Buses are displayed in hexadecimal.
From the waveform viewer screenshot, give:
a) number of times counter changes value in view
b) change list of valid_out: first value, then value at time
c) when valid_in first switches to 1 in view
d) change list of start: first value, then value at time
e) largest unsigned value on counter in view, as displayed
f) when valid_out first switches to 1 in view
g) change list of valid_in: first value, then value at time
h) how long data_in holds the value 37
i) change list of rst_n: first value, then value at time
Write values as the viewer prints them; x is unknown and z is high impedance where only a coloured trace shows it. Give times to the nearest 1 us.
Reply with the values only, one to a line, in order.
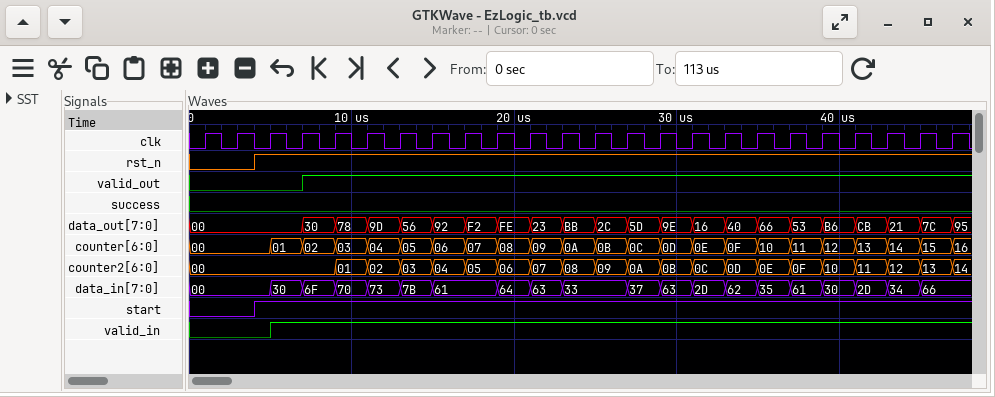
22
0, 1 at 7 us
5 us
0, 1 at 4 us
16
7 us
0, 1 at 5 us
2 us
0, 1 at 4 us
